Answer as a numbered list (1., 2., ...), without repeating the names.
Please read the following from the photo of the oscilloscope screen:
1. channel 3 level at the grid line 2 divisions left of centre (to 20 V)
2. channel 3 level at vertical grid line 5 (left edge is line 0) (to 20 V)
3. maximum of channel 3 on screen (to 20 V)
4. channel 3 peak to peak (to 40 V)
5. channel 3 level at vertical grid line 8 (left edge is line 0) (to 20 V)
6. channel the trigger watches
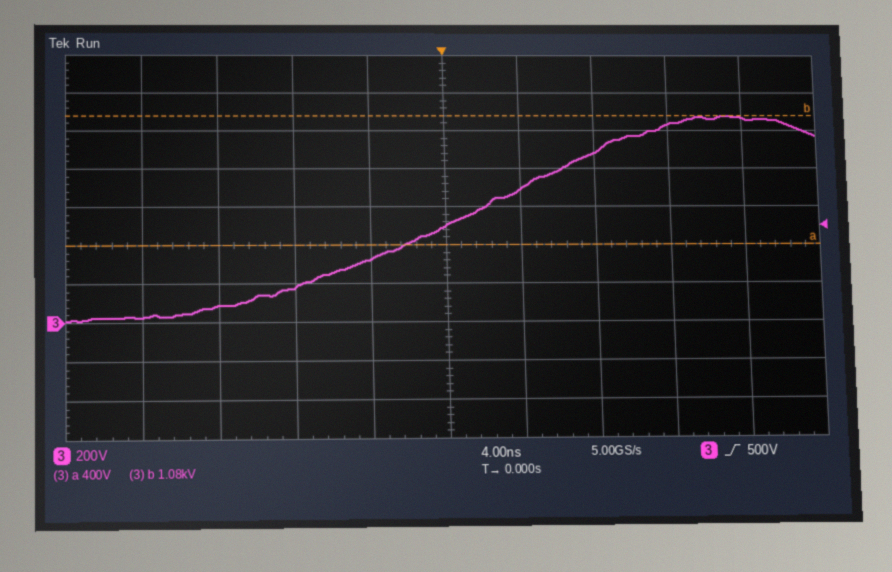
1. 180 V
2. 500 V
3. 1.08 kV
4. 1.08 kV
5. 1.04 kV
6. channel 3
